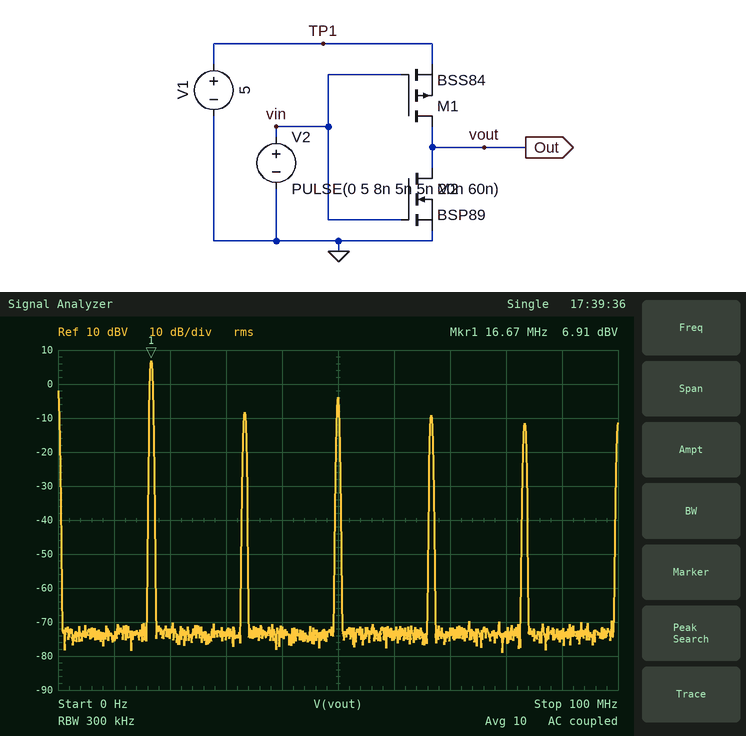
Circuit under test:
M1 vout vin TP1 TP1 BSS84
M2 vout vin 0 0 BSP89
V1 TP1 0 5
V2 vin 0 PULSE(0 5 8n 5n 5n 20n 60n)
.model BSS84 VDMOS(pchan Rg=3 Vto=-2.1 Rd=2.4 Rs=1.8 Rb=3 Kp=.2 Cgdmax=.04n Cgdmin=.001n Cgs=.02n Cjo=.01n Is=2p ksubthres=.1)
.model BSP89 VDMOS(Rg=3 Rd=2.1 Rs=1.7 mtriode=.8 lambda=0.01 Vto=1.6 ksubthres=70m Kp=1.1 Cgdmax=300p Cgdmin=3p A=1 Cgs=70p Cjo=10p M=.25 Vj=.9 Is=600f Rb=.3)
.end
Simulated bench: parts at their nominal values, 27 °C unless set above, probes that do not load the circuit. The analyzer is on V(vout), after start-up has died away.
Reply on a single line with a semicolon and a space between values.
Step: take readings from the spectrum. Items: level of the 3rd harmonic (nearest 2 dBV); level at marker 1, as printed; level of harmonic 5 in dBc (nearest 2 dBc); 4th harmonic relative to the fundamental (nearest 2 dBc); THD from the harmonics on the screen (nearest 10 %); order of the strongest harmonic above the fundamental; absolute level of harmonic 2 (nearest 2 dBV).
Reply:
-4 dBV; 6.91 dBV; -18 dBc; -16 dBc; 40 %; 3; -8 dBV
